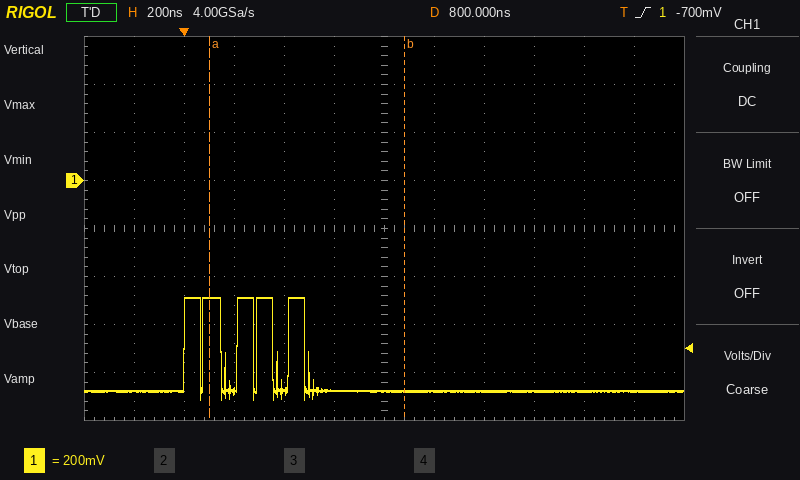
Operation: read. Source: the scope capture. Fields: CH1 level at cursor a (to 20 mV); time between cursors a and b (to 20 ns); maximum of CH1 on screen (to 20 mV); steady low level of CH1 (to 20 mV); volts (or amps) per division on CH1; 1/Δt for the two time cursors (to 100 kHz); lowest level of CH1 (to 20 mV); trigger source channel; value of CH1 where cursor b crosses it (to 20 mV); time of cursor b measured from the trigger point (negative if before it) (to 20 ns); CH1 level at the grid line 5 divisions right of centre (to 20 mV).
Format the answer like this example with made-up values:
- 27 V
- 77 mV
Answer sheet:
- -480 mV
- 780 ns
- -480 mV
- -880 mV
- 200 mV
- 1.3 MHz
- -920 mV
- CH1
- -880 mV
- +880 ns
- -880 mV
